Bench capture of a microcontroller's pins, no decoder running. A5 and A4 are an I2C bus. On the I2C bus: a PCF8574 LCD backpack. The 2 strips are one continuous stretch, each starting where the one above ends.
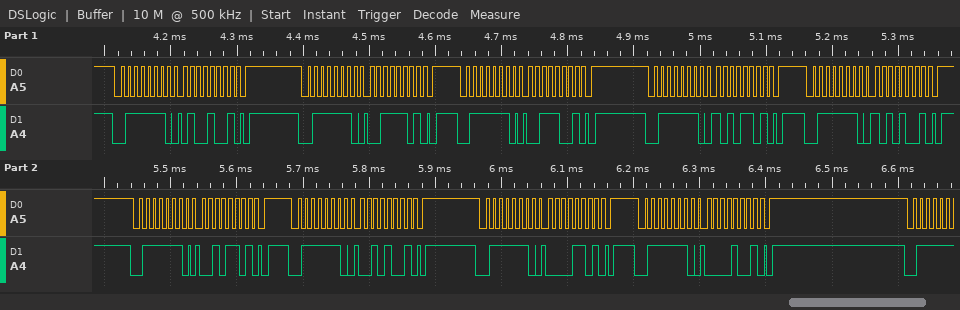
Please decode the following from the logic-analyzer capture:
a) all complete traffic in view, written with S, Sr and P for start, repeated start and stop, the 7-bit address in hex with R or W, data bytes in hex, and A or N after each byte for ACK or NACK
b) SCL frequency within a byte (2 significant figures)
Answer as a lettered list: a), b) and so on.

a) S 3FW A 49 A P S 3FW A 3D A P S 3FW A 39 A P S 3FW A AD A P S 3FW A A9 A P S 3FW A 2D A P S 3FW A 29 A P S 3FW A 0D A P S 3FW A 09 A P
b) 100 kHz
